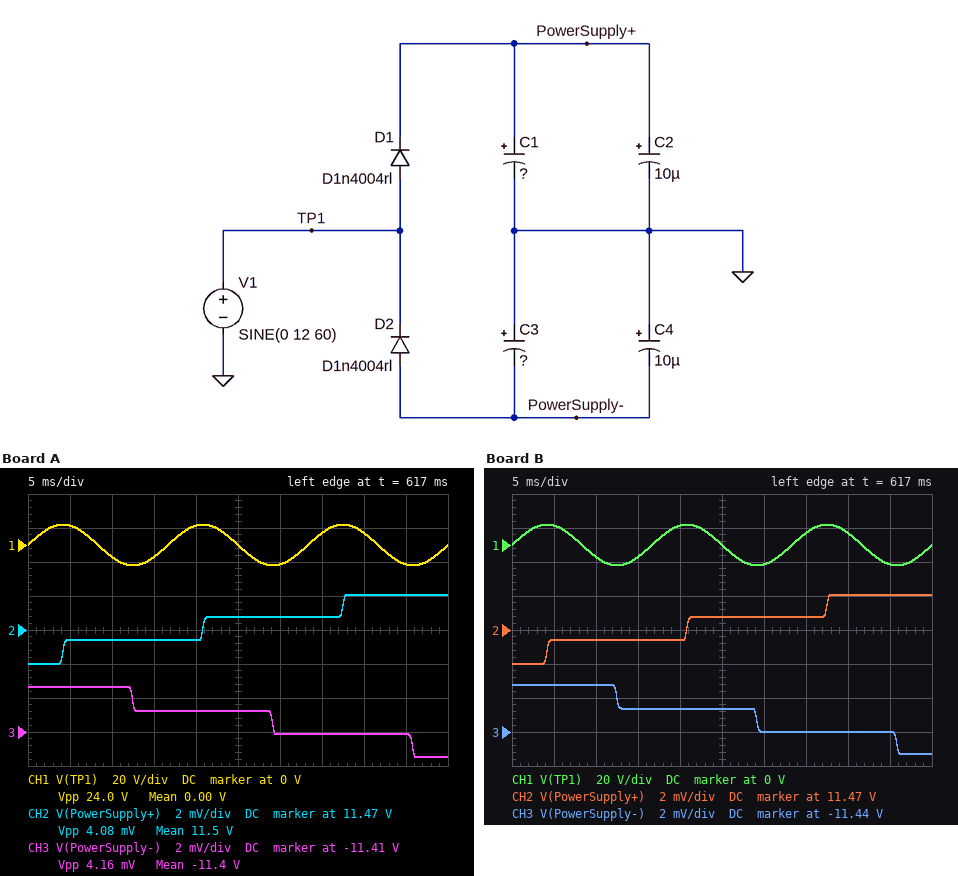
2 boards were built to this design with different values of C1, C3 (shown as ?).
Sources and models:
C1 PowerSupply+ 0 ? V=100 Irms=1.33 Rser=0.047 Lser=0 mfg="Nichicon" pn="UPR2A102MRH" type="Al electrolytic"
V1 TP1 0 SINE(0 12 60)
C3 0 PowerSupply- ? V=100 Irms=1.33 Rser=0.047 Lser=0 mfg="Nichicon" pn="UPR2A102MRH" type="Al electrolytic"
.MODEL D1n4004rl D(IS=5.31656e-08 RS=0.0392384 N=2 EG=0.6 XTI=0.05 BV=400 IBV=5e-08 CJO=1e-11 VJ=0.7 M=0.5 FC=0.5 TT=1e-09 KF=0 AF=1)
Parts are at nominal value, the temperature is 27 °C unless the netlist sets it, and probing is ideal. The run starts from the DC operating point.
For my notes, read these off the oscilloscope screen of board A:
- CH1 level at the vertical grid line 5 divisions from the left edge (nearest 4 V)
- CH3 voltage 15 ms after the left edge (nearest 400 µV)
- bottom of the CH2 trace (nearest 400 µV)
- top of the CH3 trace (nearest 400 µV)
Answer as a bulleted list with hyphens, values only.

- 0 V
- -11.4088 V
- 11.4680 V
- -11.4072 V
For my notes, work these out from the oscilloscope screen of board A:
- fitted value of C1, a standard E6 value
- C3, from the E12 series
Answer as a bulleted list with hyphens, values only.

- 470 µF
- 1.5 mF
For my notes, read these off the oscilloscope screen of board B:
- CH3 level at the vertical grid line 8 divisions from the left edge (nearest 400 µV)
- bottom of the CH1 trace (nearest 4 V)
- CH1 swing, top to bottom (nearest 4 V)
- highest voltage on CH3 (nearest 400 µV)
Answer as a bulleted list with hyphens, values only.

- -11.4420 V
- -12 V
- 24 V
- -11.4392 V
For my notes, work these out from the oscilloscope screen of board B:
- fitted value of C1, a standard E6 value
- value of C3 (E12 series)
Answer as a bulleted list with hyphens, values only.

- 470 µF
- 820 µF
